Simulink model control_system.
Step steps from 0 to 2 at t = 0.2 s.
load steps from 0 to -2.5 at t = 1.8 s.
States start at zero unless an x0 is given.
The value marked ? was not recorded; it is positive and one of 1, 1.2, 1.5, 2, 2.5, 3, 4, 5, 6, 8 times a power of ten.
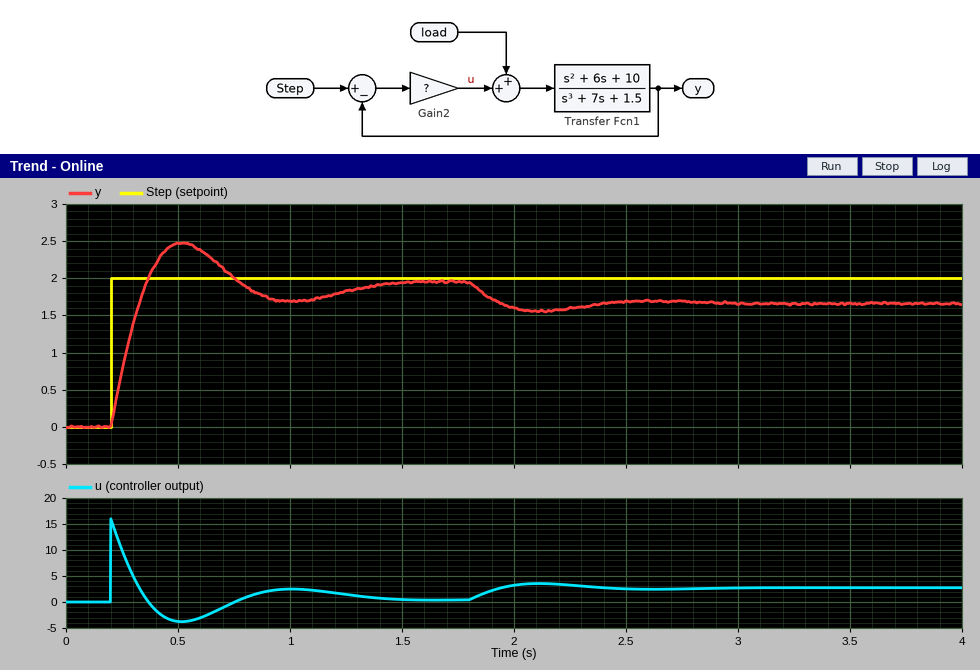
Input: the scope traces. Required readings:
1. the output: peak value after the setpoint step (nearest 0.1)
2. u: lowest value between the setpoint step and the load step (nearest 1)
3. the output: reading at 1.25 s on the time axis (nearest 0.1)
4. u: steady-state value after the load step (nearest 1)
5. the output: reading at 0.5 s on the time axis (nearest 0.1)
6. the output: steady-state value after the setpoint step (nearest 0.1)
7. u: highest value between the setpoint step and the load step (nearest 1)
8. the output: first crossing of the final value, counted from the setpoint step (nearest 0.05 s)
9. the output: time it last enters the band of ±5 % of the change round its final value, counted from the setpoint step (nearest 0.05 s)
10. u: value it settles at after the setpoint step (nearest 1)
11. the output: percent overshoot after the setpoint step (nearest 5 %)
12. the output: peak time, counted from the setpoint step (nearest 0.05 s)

2.5
-4
1.8
3
2.5
2.0
16
0.15 s
1.10 s
0
25 %
0.30 s
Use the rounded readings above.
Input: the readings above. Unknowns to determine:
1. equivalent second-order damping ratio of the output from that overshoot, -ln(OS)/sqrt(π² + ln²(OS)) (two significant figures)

0.40
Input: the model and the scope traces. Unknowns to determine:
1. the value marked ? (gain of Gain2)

8
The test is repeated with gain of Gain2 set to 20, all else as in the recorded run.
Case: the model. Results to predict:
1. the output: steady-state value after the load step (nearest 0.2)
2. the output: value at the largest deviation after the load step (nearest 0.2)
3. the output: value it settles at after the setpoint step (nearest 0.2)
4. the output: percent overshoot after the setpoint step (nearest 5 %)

1.8
1.8
2.0
15 %
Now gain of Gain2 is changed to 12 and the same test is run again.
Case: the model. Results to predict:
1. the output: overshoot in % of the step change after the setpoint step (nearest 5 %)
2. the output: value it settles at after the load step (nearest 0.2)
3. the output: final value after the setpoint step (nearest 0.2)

20 %
1.8
2.0
